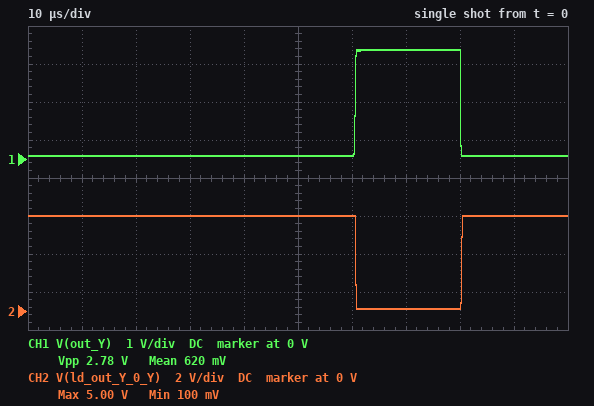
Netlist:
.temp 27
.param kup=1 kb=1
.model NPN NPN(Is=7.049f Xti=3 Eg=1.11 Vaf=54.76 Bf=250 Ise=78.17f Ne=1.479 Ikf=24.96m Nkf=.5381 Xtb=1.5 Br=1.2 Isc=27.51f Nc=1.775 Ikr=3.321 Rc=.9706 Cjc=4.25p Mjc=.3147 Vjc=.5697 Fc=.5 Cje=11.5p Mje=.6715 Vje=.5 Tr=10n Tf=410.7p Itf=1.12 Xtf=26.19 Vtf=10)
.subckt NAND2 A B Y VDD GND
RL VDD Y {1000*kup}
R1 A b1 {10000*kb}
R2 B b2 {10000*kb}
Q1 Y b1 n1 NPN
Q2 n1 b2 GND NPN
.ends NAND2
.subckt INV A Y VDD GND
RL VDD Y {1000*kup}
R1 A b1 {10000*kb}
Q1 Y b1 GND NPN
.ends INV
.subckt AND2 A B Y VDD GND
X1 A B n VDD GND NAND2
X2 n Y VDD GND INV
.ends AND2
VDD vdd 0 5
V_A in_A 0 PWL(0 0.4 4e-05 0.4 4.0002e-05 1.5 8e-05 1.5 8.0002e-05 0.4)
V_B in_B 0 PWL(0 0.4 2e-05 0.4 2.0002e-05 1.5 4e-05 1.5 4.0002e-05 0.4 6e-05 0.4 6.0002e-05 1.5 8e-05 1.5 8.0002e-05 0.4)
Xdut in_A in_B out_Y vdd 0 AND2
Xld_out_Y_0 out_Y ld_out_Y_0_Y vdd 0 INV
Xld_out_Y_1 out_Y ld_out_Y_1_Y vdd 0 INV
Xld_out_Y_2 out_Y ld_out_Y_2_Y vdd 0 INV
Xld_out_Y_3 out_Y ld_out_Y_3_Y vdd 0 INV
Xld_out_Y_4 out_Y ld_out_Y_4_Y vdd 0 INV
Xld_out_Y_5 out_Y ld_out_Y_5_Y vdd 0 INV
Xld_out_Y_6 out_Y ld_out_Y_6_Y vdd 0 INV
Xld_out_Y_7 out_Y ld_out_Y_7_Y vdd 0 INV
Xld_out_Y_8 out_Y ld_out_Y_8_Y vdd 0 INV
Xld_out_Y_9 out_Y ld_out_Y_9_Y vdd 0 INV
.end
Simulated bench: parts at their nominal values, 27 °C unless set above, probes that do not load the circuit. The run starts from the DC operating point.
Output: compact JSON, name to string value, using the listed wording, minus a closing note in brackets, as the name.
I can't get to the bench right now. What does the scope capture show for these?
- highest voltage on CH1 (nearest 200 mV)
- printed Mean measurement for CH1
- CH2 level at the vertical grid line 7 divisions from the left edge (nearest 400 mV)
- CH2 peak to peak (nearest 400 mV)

{"highest voltage on CH1": "2.8 V", "printed Mean measurement for CH1": "620 mV", "CH2 level at the vertical grid line 7 divisions from the left edge": "0 V", "CH2 peak to peak": "4.8 V"}
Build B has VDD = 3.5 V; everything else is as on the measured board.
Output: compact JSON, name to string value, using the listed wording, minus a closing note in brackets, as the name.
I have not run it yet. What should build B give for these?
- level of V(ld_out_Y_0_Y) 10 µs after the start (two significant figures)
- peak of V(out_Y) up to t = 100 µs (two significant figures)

{"level of V(ld_out_Y_0_Y) 10 µs after the start": "3.5 V", "peak of V(out_Y) up to t = 100 µs": "2.1 V"}
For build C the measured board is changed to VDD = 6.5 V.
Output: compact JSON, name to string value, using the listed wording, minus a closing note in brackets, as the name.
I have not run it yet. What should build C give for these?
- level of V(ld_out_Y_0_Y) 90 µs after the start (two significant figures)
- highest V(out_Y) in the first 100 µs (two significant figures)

{"level of V(ld_out_Y_0_Y) 90 µs after the start": "6.5 V", "highest V(out_Y) in the first 100 µs": "3.6 V"}
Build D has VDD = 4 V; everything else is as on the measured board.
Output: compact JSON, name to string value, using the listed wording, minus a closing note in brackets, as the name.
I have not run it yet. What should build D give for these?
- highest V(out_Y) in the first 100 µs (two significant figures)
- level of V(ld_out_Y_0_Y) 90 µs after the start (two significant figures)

{"highest V(out_Y) in the first 100 µs": "2.4 V", "level of V(ld_out_Y_0_Y) 90 µs after the start": "4.0 V"}
